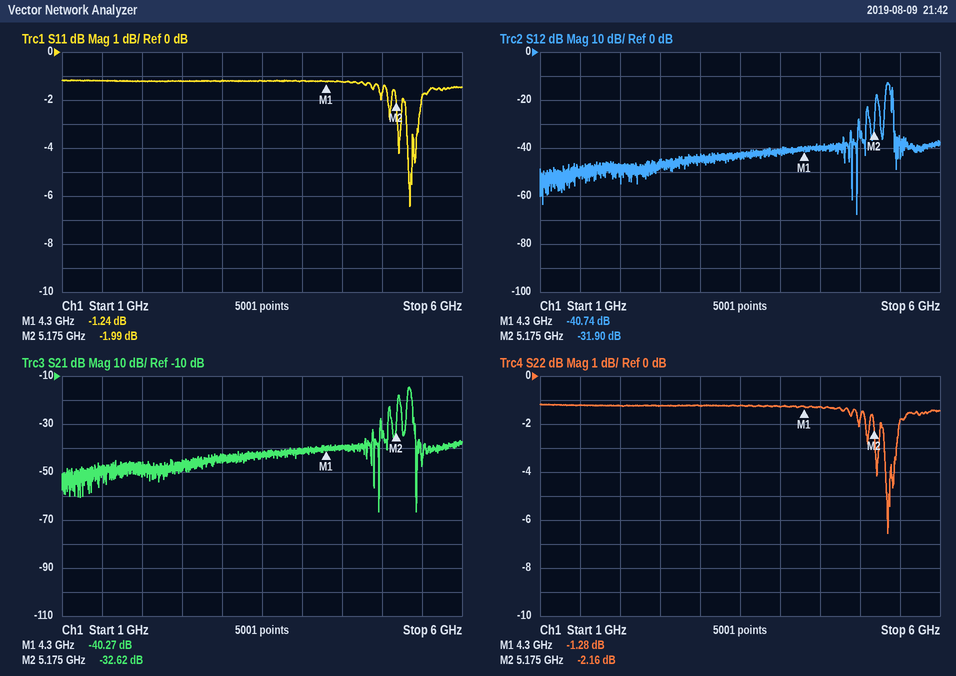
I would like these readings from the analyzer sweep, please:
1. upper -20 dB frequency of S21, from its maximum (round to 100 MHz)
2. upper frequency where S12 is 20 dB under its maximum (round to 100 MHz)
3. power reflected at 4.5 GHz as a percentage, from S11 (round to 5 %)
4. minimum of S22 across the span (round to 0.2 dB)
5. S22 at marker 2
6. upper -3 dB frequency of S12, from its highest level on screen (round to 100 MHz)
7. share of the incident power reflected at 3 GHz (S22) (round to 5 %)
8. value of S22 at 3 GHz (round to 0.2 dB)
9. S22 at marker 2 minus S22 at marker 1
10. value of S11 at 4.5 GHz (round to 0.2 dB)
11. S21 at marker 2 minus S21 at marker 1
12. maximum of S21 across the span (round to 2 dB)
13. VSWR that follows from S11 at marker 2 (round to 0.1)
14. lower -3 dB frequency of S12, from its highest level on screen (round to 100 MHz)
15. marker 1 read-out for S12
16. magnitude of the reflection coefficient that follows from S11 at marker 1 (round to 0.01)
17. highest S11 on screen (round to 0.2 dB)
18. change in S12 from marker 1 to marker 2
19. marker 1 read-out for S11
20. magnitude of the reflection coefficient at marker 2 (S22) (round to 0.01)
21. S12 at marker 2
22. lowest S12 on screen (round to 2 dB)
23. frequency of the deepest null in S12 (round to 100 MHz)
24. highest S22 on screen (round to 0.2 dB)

5.4 GHz
5.4 GHz
75 %
-6.6 dB
-2.16 dB
5.4 GHz
75 %
-1.2 dB
-0.88 dB
-1.2 dB
7.65 dB
-14 dB
8.8
5.3 GHz
-40.74 dB
0.87
-1.2 dB
8.84 dB
-1.24 dB
0.78
-31.90 dB
-68 dB
5.0 GHz
-1.2 dB
